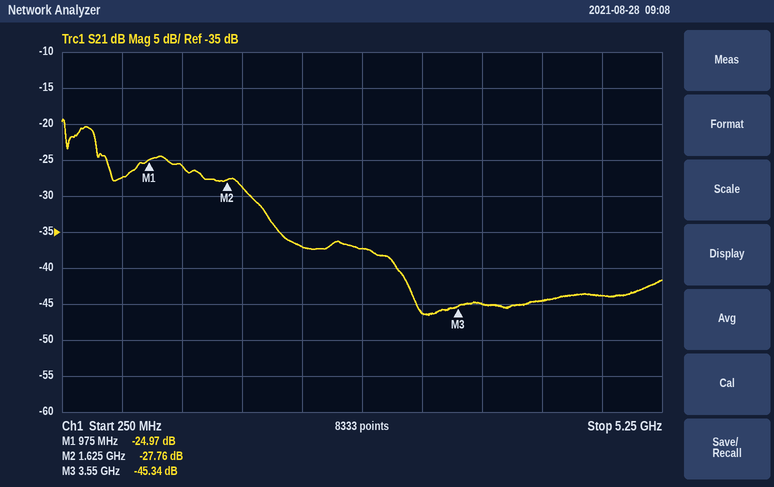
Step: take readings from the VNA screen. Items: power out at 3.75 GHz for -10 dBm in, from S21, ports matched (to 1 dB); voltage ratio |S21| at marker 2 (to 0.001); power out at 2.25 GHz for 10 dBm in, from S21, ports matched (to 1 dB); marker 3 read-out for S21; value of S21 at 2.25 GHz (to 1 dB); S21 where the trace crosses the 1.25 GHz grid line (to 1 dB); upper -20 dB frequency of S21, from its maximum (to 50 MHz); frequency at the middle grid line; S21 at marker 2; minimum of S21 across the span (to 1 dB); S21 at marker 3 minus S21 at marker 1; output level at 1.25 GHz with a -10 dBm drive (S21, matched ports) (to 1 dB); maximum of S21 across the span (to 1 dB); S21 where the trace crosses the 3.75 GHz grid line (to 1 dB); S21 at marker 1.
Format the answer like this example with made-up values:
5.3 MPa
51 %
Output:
-55 dBm
0.041
-27 dBm
-45.34 dB
-37 dB
-26 dB
3.00 GHz
2.75 GHz
-27.76 dB
-47 dB
-20.37 dB
-36 dBm
-19 dB
-45 dB
-24.97 dB
